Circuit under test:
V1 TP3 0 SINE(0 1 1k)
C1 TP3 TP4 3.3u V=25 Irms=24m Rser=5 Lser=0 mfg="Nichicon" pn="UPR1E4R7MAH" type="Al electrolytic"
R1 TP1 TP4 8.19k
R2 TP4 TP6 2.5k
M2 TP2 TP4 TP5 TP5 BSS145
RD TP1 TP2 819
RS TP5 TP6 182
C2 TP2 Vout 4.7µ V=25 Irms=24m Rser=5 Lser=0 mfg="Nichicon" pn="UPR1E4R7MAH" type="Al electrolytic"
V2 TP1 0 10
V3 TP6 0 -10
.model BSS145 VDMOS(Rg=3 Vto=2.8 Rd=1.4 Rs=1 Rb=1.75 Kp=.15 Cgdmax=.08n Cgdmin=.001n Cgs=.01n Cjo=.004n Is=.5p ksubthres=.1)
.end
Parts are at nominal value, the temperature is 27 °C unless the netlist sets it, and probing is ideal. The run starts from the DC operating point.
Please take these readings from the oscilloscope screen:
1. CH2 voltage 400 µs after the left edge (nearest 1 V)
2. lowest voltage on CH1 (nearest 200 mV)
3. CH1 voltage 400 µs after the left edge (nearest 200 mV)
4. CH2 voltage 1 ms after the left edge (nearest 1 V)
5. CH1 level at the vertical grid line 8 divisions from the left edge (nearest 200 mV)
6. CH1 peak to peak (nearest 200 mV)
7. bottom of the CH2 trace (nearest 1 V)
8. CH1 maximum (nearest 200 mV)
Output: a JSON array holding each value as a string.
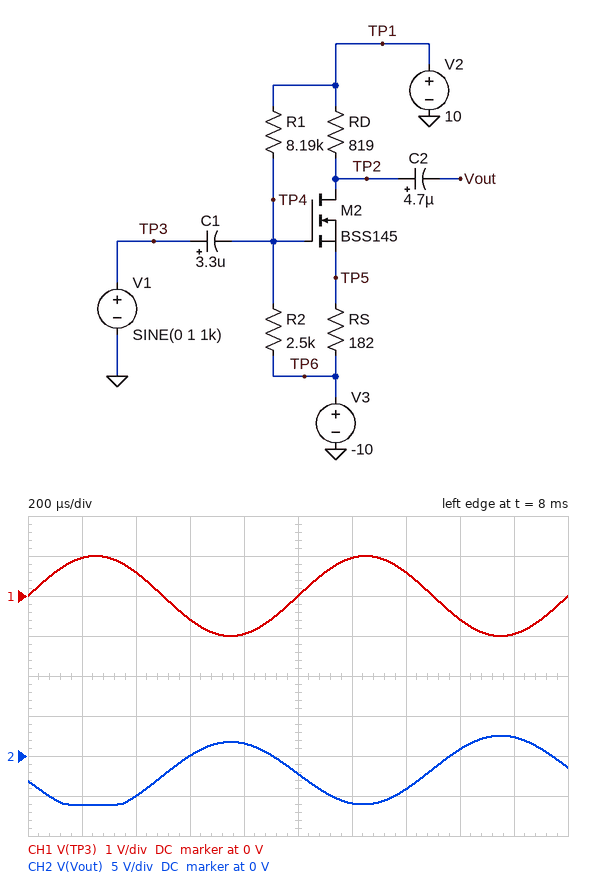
["-5 V", "-1.0 V", "600 mV", "-2 V", "-600 mV", "2.0 V", "-6 V", "1.0 V"]
